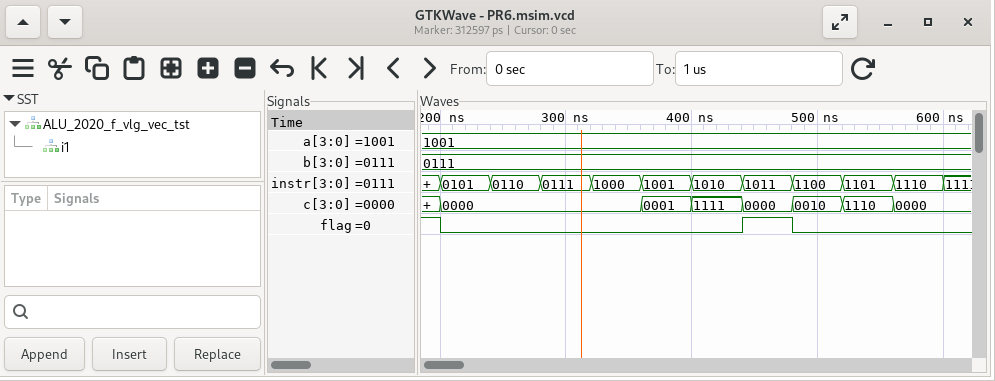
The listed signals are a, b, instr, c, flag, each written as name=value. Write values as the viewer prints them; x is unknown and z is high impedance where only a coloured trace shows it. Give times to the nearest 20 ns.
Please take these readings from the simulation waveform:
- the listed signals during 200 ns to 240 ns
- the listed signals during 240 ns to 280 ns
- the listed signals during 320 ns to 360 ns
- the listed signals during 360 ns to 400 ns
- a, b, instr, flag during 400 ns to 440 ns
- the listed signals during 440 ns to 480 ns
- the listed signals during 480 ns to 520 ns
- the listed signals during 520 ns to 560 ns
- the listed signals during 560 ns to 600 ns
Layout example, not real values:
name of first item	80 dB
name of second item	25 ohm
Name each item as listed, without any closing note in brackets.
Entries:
the listed signals during 200 ns to 240 ns	a=1001, b=0111, instr=0101, c=0000, flag=0
the listed signals during 240 ns to 280 ns	a=1001, b=0111, instr=0110, c=0000, flag=0
the listed signals during 320 ns to 360 ns	a=1001, b=0111, instr=1000, c=0000, flag=0
the listed signals during 360 ns to 400 ns	a=1001, b=0111, instr=1001, c=0001, flag=0
a, b, instr, flag during 400 ns to 440 ns	a=1001, b=0111, instr=1010, flag=0
the listed signals during 440 ns to 480 ns	a=1001, b=0111, instr=1011, c=0000, flag=1
the listed signals during 480 ns to 520 ns	a=1001, b=0111, instr=1100, c=0010, flag=0
the listed signals during 520 ns to 560 ns	a=1001, b=0111, instr=1101, c=1110, flag=0
the listed signals during 560 ns to 600 ns	a=1001, b=0111, instr=1110, c=0000, flag=0
